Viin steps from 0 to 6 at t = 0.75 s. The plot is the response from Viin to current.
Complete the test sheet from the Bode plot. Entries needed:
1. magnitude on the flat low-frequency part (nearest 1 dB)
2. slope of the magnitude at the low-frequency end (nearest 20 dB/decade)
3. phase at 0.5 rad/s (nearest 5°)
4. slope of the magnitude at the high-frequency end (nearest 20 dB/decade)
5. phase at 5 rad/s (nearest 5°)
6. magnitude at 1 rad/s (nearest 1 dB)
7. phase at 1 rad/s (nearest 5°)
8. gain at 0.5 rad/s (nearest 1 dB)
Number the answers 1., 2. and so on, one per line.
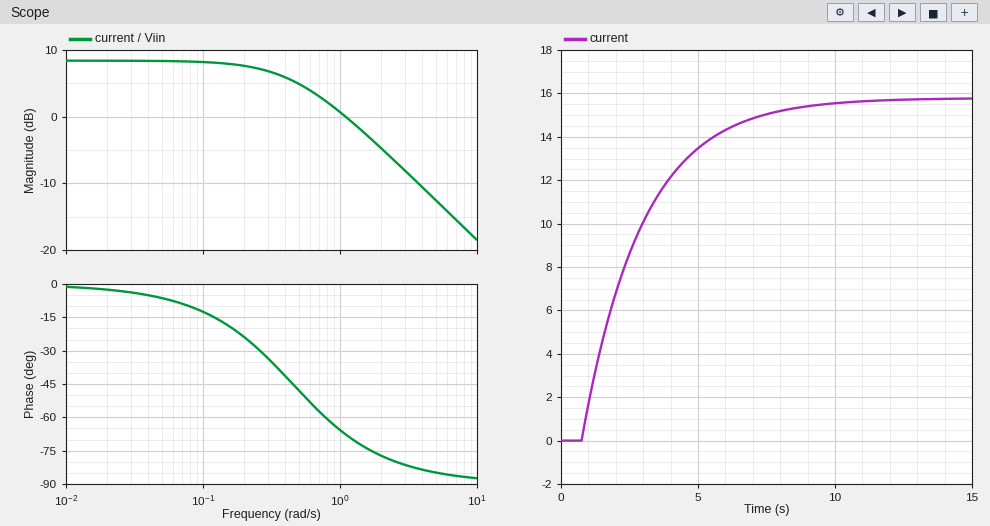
1. 8 dB
2. 0 dB/decade
3. -50°
4. -20 dB/decade
5. -85°
6. 1 dB
7. -65°
8. 5 dB
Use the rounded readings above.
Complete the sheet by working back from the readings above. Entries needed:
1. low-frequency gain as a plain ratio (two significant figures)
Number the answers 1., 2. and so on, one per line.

1. 2.5
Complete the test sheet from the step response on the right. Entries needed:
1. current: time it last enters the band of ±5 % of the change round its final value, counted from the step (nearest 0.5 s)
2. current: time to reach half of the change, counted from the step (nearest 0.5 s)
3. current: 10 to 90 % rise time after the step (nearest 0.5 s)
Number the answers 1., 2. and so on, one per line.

1. 6.5 s
2. 1.5 s
3. 5.0 s
